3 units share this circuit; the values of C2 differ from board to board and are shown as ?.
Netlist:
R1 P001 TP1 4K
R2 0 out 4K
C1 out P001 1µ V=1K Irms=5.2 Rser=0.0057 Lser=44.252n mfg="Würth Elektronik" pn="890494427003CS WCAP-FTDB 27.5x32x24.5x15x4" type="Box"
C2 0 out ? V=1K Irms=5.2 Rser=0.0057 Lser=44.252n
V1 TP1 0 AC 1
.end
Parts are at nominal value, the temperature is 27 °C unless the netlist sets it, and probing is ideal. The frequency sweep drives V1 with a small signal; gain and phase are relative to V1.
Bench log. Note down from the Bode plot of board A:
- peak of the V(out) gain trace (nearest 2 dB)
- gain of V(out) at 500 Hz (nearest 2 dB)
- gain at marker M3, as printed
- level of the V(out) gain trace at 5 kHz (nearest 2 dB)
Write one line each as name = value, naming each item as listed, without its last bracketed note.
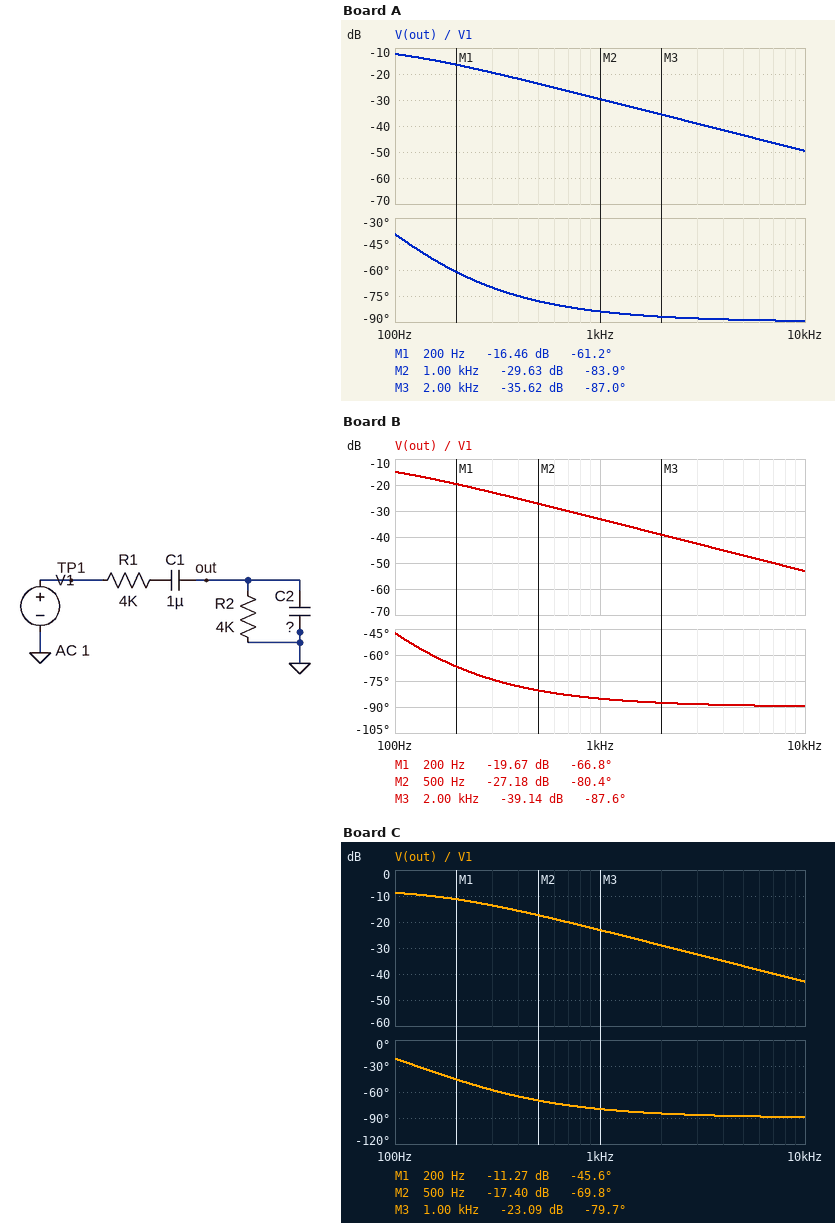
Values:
peak of the V(out) gain trace = -12 dB
gain of V(out) at 500 Hz = -24 dB
gain at marker M3, as printed = -35.62 dB
level of the V(out) gain trace at 5 kHz = -44 dB
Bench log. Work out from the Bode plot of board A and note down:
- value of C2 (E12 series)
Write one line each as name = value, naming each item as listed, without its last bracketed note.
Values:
value of C2 = 1.2 µF
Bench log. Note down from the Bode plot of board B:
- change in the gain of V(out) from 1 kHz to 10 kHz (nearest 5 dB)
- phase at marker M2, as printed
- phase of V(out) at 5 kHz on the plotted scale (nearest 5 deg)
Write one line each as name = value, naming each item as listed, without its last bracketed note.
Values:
change in the gain of V(out) from 1 kHz to 10 kHz = -20 dB
phase at marker M2, as printed = -80.4 deg
phase of V(out) at 5 kHz on the plotted scale = -90 deg
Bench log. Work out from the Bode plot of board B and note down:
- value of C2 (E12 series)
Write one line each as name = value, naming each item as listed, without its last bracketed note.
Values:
value of C2 = 1.8 µF
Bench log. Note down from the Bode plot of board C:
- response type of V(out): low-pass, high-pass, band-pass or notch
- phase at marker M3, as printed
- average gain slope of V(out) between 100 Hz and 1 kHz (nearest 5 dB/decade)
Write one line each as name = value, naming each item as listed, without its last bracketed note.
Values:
response type of V(out): low-pass, high-pass, band-pass or notch = low-pass
phase at marker M3, as printed = -79.7 deg
average gain slope of V(out) between 100 Hz and 1 kHz = -15 dB/decade
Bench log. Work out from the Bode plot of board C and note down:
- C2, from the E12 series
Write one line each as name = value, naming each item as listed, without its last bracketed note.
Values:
C2, from the E12 series = 560 nF
